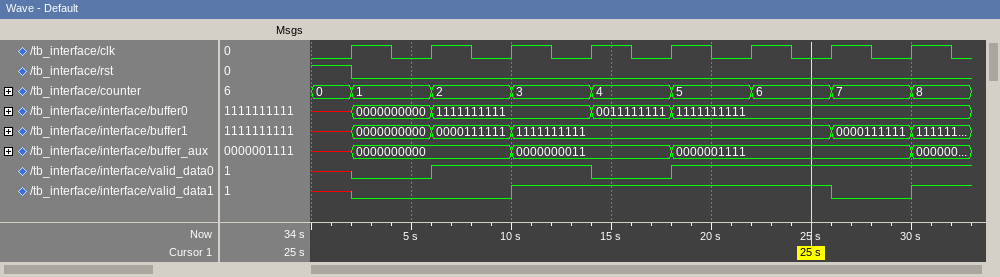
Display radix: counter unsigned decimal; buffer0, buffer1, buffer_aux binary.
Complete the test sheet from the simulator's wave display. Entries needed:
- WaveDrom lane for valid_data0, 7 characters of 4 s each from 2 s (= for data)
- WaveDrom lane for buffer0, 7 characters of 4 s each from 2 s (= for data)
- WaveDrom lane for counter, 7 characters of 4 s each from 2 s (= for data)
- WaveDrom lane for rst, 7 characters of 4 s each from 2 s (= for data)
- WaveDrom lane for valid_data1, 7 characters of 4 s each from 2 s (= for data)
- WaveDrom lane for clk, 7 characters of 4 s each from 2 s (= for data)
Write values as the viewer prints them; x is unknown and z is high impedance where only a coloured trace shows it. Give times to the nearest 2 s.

{name: 'valid_data0', wave: '01.01..'}
{name: 'buffer0', wave: '==.==..', data: '0000000000 1111111111 0011111111 1111111111'}
{name: 'counter', wave: '=======', data: '1 2 3 4 5 6 7'}
{name: 'rst', wave: '0......'}
{name: 'valid_data1', wave: '0.1...0'}
{name: 'clk', wave: 'p......'}
